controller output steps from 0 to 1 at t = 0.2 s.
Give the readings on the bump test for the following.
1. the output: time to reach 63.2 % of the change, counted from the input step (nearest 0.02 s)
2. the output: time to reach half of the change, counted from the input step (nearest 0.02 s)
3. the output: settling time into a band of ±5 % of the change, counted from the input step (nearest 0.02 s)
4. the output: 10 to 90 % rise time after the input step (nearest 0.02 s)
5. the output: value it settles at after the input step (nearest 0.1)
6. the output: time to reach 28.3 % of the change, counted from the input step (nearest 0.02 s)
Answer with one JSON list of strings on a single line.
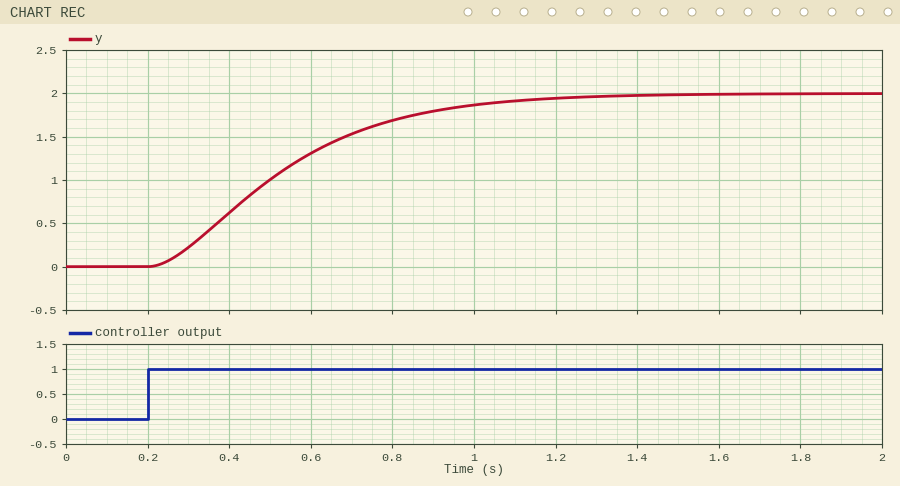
["0.38 s", "0.30 s", "0.86 s", "0.62 s", "2.0", "0.18 s"]
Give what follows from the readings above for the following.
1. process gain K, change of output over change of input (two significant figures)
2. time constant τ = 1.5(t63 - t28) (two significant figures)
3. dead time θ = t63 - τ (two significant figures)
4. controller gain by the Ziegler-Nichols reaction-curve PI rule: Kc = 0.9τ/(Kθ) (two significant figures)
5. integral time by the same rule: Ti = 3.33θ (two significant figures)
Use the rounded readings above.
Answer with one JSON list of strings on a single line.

["2.0", "0.30 s", "0.080 s", "1.7", "0.27 s"]
